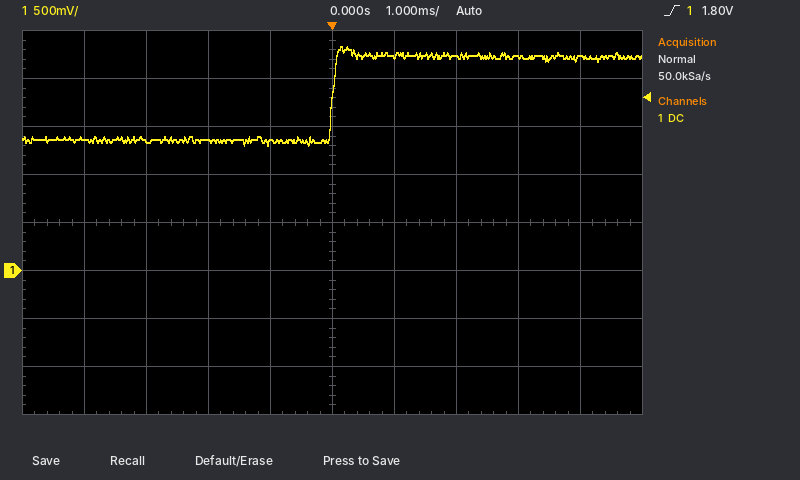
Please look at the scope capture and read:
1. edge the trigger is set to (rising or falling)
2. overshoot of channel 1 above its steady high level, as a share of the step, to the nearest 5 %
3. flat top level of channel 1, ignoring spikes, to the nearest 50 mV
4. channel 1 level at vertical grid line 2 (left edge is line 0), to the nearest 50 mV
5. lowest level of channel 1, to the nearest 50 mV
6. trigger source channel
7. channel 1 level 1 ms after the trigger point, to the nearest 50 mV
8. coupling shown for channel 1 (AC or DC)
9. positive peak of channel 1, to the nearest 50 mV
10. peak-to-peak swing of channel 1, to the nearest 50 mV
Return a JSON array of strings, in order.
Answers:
["rising", "10 %", "2.25 V", "1.35 V", "1.30 V", "channel 1", "2.25 V", "DC", "2.35 V", "1.05 V"]
